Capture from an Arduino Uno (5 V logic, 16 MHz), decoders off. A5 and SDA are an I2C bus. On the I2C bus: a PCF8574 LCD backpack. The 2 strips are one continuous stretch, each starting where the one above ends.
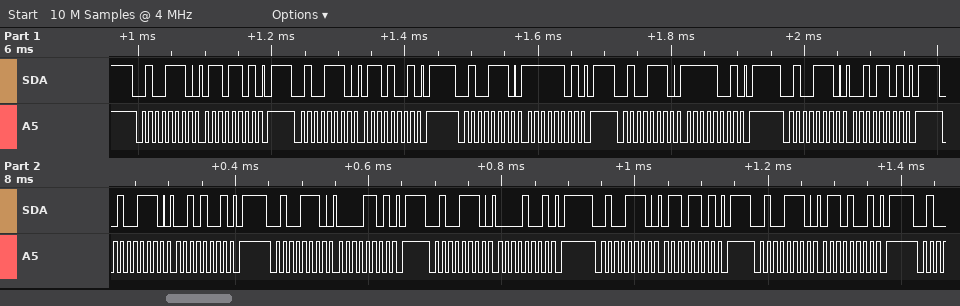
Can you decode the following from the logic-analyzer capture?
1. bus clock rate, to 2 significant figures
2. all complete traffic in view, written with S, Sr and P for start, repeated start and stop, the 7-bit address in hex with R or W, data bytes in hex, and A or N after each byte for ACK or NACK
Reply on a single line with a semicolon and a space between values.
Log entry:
100 kHz; S 27W A 6D A P S 27W A 69 A P S 27W A FD A P S 27W A F9 A P S 27W A 2D A P S 27W A 29 A P S 27W A 0D A P S 27W A 09 A P S 27W A 6D A P S 27W A 69 A P
